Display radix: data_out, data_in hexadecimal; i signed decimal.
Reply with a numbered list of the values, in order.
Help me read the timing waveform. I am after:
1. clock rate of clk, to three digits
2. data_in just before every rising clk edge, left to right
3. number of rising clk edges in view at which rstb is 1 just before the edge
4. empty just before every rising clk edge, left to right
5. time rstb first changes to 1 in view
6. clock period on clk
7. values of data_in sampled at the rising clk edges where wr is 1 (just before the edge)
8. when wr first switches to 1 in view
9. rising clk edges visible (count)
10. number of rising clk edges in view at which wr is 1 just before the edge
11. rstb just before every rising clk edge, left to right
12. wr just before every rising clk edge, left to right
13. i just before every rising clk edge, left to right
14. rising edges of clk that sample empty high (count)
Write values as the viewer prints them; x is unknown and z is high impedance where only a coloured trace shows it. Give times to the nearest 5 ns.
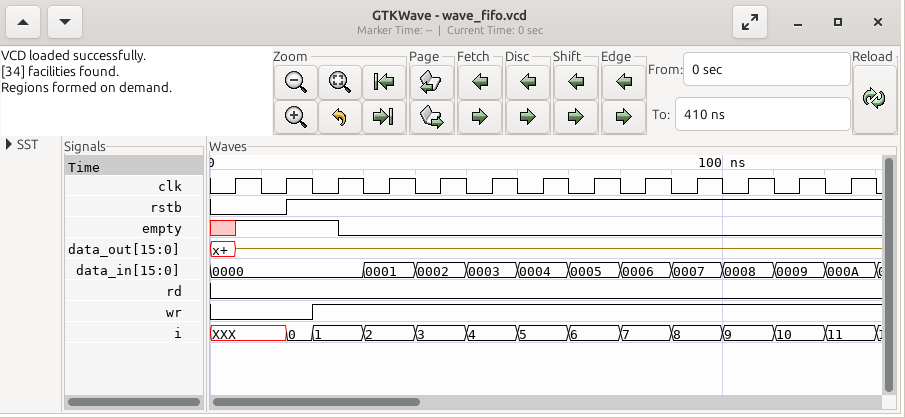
1. 100 MHz
2. 0000, 0000, 0000, 0001, 0002, 0003, 0004, 0005, 0006, 0007, 0008, 0009, 000A
3. 11
4. x 1 1 0 0 0 0 0 0 0 0 0 0
5. 15 ns
6. 10 ns
7. 0000, 0001, 0002, 0003, 0004, 0005, 0006, 0007, 0008, 0009, 000A
8. 20 ns
9. 13
10. 11
11. 0 0 1 1 1 1 1 1 1 1 1 1 1
12. 0 0 1 1 1 1 1 1 1 1 1 1 1
13. XXX, XXX, 1, 2, 3, 4, 5, 6, 7, 8, 9, 10, 11
14. 2
